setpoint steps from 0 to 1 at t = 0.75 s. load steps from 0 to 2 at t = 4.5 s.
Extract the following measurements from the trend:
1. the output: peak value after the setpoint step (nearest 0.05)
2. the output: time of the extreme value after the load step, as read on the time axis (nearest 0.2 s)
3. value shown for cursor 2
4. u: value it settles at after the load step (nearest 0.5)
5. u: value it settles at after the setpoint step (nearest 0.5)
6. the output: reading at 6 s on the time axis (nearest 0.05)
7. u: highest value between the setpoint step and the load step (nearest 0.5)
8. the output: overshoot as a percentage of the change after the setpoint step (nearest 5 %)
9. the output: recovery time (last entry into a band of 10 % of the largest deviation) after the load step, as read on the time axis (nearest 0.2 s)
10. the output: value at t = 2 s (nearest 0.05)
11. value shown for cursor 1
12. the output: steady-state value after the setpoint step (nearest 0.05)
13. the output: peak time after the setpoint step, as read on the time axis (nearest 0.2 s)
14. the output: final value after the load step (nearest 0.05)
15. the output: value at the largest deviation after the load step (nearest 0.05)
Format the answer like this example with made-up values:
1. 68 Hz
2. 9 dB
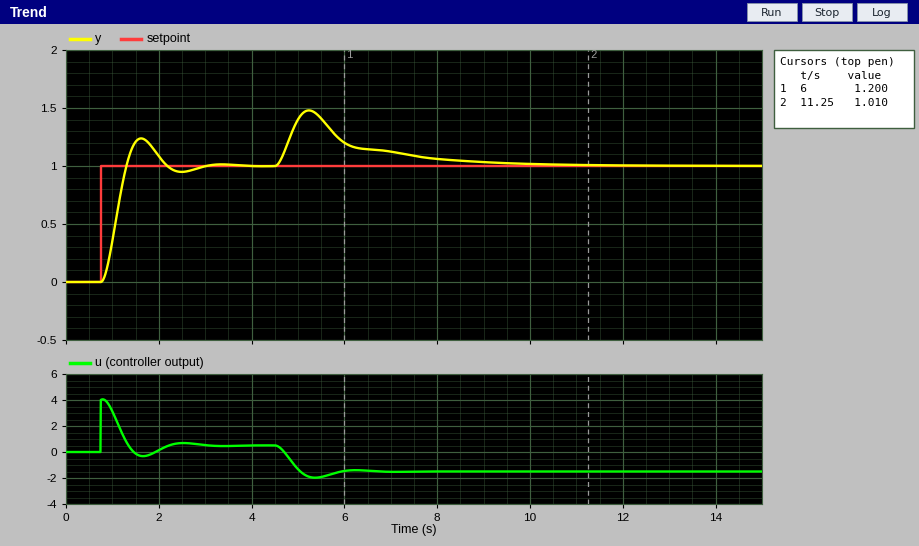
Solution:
1. 1.25
2. 5.2 s
3. 1.010
4. -1.5
5. 0.5
6. 1.20
7. 4.0
8. 25 %
9. 8.4 s
10. 1.10
11. 1.200
12. 1.00
13. 1.6 s
14. 1.00
15. 1.50
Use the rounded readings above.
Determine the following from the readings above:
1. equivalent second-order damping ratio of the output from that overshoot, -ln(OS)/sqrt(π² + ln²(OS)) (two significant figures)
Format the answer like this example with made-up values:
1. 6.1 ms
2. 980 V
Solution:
1. 0.40
